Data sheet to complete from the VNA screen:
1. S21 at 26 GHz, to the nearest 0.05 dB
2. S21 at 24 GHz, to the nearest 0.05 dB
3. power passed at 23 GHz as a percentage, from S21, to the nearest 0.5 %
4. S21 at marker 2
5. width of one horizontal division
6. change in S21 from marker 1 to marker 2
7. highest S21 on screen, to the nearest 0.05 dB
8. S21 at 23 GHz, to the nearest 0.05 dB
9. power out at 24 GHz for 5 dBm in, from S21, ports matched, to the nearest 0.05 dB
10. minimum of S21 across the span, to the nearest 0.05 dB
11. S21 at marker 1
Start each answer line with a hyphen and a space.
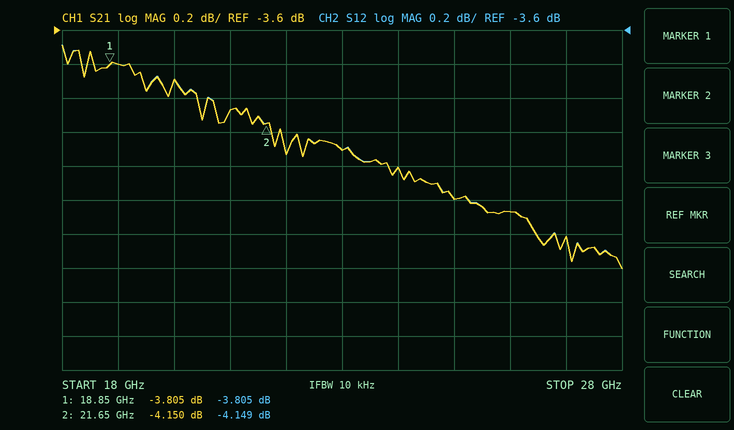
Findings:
- -4.65 dB
- -4.40 dB
- 37.0 %
- -4.150 dB
- 1 GHz
- -0.345 dB
- -3.70 dB
- -4.30 dB
- 0.60 dBm
- -5.00 dB
- -3.805 dB
